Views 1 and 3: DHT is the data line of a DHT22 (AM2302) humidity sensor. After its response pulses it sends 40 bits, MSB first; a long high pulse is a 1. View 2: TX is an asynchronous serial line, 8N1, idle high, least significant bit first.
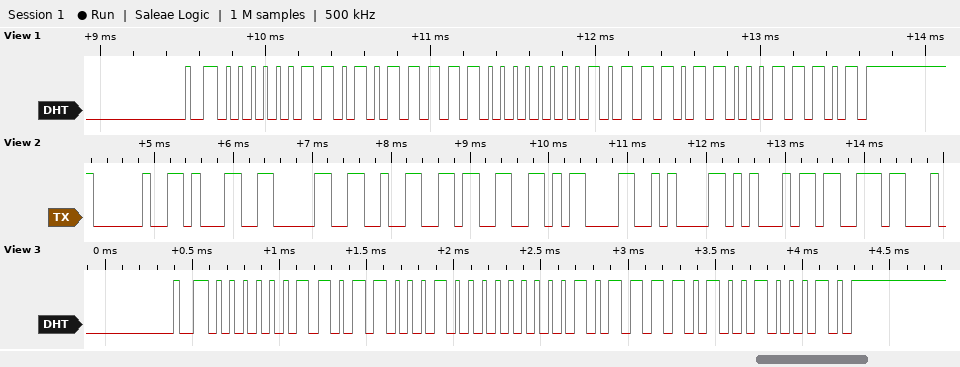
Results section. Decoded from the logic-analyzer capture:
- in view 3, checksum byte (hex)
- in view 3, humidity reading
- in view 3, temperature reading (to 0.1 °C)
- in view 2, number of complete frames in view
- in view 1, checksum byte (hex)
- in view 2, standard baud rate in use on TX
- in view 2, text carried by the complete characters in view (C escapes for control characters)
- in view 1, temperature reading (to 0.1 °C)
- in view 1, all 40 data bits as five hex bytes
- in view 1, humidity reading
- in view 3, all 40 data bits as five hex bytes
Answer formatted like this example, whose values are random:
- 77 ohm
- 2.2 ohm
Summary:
- 0x22
- 86.6 %
- 18.9 °C
- 9
- 0x1D
- 9600 baud
- " 1023\r\nEs"
- 18.7 °C
- 03 5F 00 BB 1D
- 86.3 %
- 03 62 00 BD 22
